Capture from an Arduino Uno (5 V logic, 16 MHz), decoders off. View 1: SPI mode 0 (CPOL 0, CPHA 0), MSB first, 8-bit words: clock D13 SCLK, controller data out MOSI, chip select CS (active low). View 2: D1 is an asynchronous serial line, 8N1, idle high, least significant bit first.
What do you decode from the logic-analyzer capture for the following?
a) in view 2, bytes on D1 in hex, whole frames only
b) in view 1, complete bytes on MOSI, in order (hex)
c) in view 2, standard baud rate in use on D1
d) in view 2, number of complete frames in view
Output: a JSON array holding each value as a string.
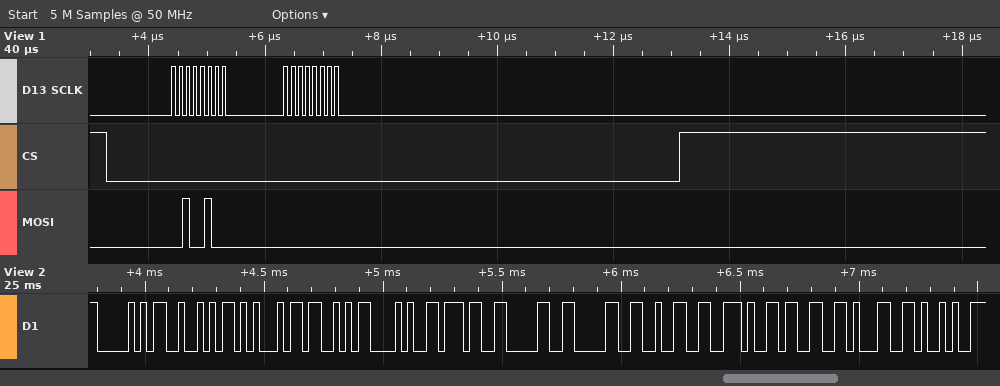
["0x50 0x52 0x45 0x53 0x28 0x37 0x30 0x30 0x32 0x2E 0x33 0x31 0x29", "0x24 0x00", "38400 baud", "13"]
